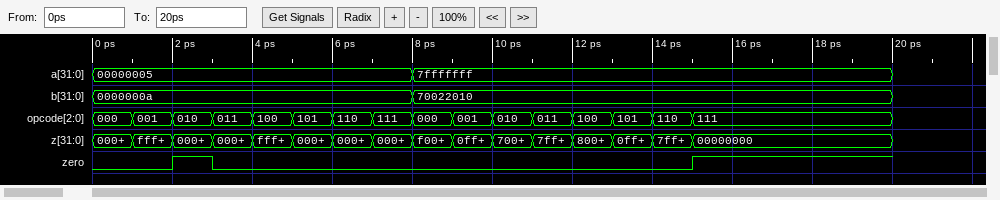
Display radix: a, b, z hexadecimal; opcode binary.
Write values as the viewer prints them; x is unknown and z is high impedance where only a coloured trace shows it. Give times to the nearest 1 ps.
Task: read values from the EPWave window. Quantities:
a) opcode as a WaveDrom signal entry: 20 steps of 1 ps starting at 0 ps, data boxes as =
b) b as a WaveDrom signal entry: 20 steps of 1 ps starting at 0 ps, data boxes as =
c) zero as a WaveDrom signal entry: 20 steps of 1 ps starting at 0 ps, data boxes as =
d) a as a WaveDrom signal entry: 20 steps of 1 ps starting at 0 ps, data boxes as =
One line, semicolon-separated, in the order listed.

{name: 'opcode', wave: '================....', data: '000 001 010 011 100 101 110 111 000 001 010 011 100 101 110 111'}; {name: 'b', wave: '=.......=...........', data: '0000000a 70022010'}; {name: 'zero', wave: '0.10...........1....'}; {name: 'a', wave: '=.......=...........', data: '00000005 7fffffff'}
